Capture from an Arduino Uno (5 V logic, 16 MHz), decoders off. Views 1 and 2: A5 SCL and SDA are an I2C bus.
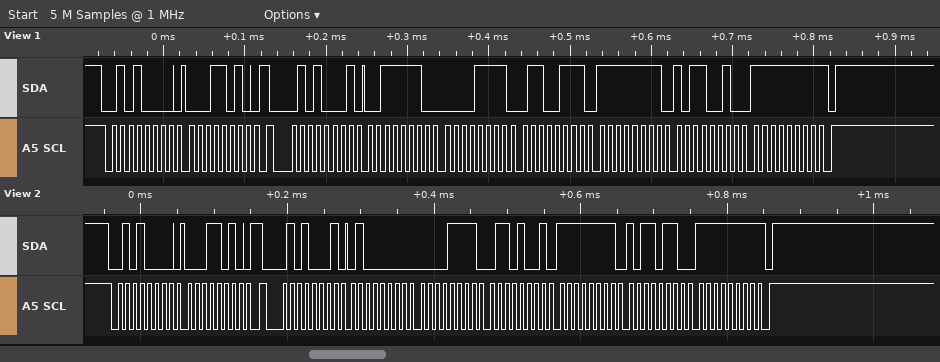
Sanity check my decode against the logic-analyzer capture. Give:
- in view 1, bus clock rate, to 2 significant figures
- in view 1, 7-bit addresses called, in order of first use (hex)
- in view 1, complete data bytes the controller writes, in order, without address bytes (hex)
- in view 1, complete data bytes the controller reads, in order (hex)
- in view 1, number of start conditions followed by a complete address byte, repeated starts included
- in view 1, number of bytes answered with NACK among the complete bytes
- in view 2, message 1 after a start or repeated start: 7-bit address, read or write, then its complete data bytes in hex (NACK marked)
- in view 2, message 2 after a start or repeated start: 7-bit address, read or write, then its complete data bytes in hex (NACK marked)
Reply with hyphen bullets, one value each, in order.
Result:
- 100 kHz
- 0x28
- 1A
- 3E 0F 67 FF B2 FF
- 2
- 1
- 0x28 write: 1A
- 0x28 read: 40 0F 69 FF B6 FF NACK
